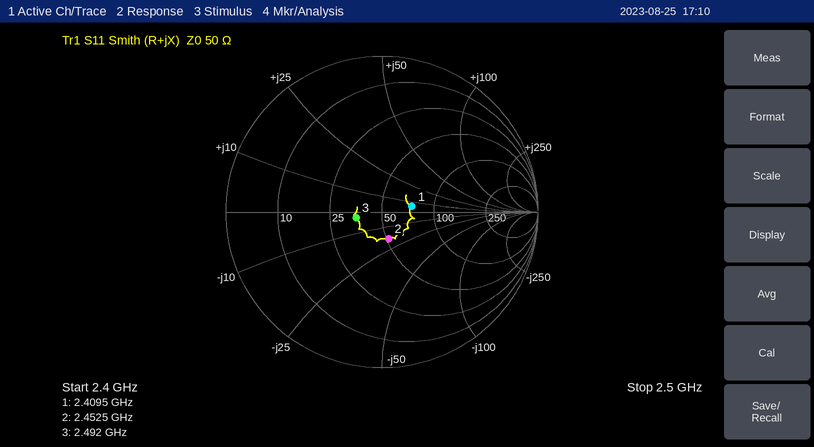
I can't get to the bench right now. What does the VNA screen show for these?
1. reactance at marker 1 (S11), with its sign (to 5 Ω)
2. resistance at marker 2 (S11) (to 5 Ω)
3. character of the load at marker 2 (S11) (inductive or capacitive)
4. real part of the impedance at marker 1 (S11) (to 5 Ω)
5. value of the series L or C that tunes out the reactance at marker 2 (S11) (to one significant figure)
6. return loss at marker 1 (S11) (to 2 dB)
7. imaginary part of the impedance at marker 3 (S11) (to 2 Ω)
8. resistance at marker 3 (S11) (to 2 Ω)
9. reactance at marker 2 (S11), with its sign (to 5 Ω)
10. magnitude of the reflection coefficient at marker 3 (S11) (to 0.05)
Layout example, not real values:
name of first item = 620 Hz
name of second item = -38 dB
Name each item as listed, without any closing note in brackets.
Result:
reactance at marker 1 (S11), with its sign = +5 Ω
resistance at marker 2 (S11) = 50 Ω
character of the load at marker 2 (S11) = capacitive
real part of the impedance at marker 1 (S11) = 75 Ω
value of the series L or C that tunes out the reactance at marker 2 (S11) = 1 nH
return loss at marker 1 (S11) = 14 dB
imaginary part of the impedance at marker 3 (S11) = -2 Ω
resistance at marker 3 (S11) = 36 Ω
reactance at marker 2 (S11), with its sign = -20 Ω
magnitude of the reflection coefficient at marker 3 (S11) = 0.15
